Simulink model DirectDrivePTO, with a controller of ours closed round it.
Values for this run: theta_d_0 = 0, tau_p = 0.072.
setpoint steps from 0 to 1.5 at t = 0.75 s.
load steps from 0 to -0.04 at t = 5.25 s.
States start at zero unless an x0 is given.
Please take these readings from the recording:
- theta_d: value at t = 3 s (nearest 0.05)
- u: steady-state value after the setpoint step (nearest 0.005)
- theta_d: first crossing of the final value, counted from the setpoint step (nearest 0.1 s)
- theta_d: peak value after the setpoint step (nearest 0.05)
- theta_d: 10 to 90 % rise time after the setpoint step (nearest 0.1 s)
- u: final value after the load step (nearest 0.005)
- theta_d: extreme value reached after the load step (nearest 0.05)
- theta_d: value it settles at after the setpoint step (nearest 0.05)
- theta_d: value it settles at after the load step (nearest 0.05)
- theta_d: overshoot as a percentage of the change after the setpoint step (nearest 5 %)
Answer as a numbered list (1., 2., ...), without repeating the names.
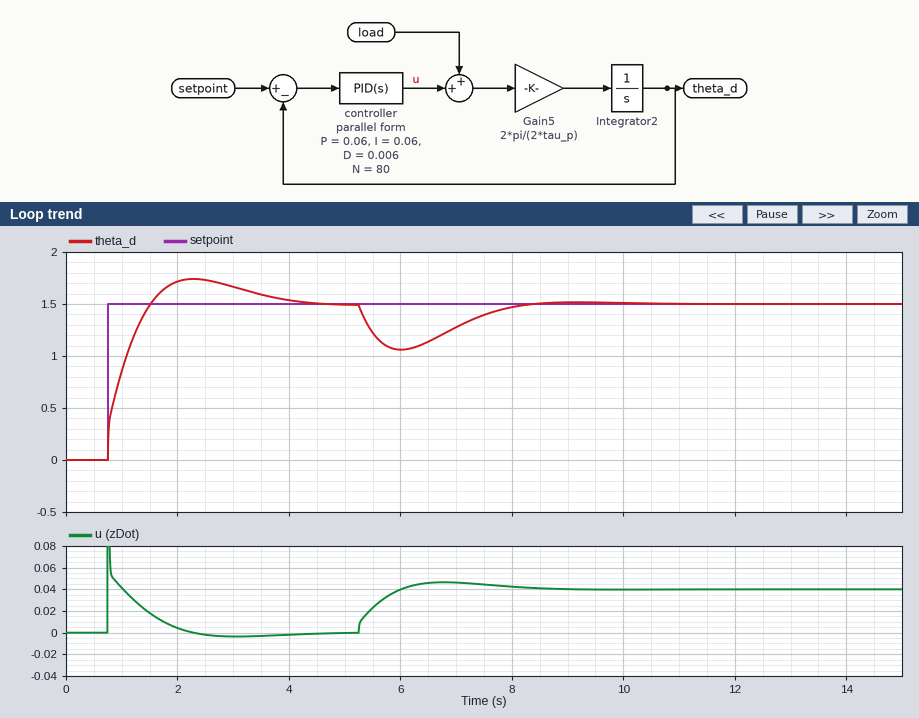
1. 1.65
2. 0.000
3. 0.8 s
4. 1.75
5. 0.6 s
6. 0.040
7. 1.05
8. 1.50
9. 1.50
10. 15 %
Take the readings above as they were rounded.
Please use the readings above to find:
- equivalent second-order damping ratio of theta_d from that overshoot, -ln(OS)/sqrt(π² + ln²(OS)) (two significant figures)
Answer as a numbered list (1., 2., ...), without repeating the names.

1. 0.52
